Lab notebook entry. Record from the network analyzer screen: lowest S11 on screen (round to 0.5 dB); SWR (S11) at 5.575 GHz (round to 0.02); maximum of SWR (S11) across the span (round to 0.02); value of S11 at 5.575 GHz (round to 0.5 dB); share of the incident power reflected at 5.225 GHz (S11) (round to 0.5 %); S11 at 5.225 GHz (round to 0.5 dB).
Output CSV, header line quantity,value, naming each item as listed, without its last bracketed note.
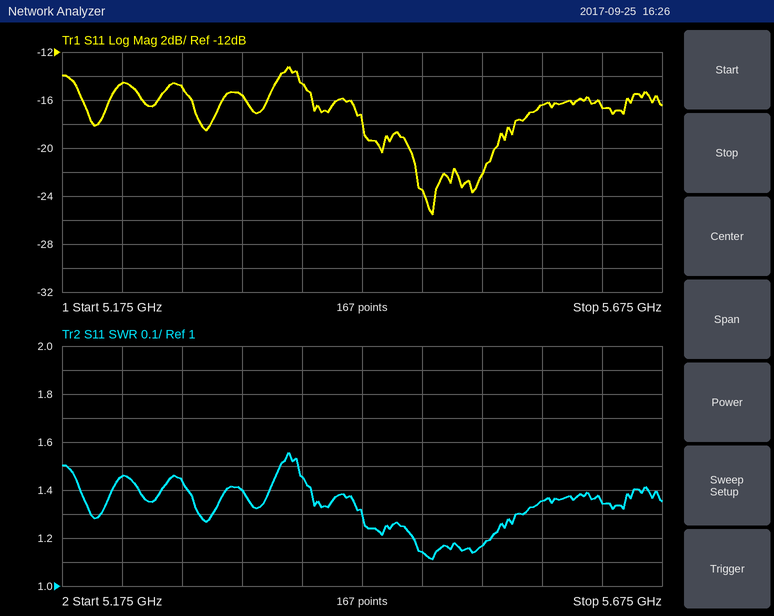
quantity,value
lowest S11 on screen,-25.5 dB
SWR (S11) at 5.575 GHz,1.36
maximum of SWR (S11) across the span,1.56
value of S11 at 5.575 GHz,-16.5 dB
share of the incident power reflected at 5.225 GHz (S11),3.5 %
S11 at 5.225 GHz,-14.5 dB
